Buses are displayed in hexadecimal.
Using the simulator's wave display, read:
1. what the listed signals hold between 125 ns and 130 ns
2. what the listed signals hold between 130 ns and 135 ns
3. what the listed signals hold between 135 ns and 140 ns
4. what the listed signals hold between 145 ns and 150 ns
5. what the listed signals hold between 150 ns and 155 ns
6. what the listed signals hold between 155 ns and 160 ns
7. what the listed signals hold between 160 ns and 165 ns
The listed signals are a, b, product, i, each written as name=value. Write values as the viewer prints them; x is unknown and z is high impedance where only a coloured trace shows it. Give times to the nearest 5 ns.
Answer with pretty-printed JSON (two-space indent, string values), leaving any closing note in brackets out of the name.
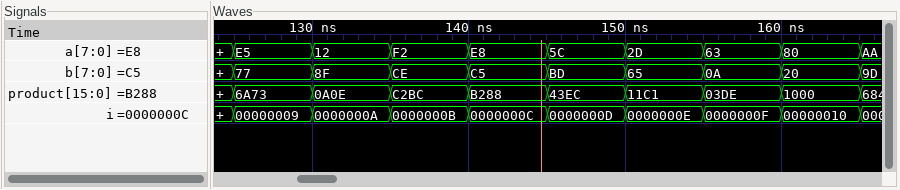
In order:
{
  "what the listed signals hold between 125 ns and 130 ns": "a=E5, b=77, product=6A73, i=00000009",
  "what the listed signals hold between 130 ns and 135 ns": "a=12, b=8F, product=0A0E, i=0000000A",
  "what the listed signals hold between 135 ns and 140 ns": "a=F2, b=CE, product=C2BC, i=0000000B",
  "what the listed signals hold between 145 ns and 150 ns": "a=5C, b=BD, product=43EC, i=0000000D",
  "what the listed signals hold between 150 ns and 155 ns": "a=2D, b=65, product=11C1, i=0000000E",
  "what the listed signals hold between 155 ns and 160 ns": "a=63, b=0A, product=03DE, i=0000000F",
  "what the listed signals hold between 160 ns and 165 ns": "a=80, b=20, product=1000, i=00000010"
}
